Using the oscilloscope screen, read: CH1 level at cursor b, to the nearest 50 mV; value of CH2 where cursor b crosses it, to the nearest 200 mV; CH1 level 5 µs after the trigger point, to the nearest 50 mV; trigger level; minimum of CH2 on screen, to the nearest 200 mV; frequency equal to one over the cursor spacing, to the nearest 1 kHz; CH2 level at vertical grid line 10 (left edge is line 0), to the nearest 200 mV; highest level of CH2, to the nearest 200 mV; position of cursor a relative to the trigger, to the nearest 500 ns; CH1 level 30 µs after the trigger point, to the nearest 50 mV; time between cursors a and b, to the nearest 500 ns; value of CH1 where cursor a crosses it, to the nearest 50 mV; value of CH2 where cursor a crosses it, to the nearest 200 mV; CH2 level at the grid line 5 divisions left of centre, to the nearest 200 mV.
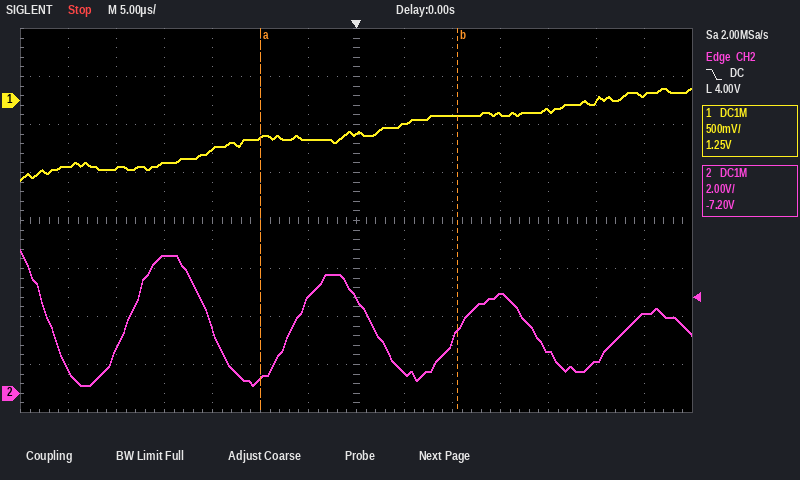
-150 mV
2.6 V
-250 mV
4.00 V
400 mV
49 kHz
4.2 V
6.0 V
-10.0 µs
50 mV
20.5 µs
-400 mV
600 mV
1.8 V
